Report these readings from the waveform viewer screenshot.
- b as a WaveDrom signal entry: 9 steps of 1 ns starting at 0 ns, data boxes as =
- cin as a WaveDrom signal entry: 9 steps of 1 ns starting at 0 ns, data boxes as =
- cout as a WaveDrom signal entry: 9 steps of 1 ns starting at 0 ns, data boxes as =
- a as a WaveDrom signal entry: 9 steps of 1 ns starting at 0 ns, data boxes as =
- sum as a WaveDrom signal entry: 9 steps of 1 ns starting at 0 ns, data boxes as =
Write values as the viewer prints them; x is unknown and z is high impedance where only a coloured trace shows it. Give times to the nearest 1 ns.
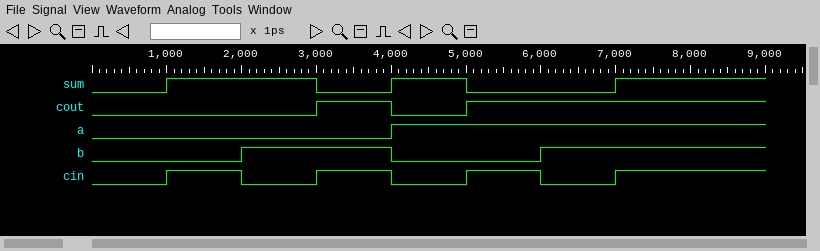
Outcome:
{name: 'b', wave: '0.1.0.1..'}
{name: 'cin', wave: '01010101.'}
{name: 'cout', wave: '0..101...'}
{name: 'a', wave: '0...1....'}
{name: 'sum', wave: '01.010.1.'}
